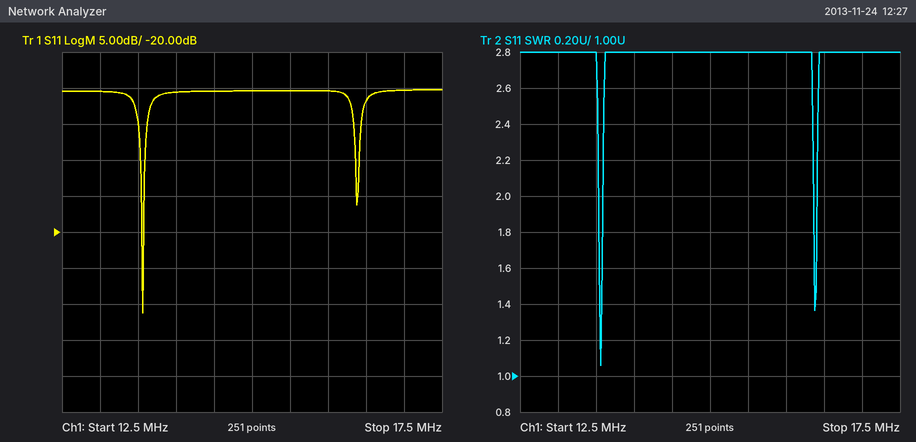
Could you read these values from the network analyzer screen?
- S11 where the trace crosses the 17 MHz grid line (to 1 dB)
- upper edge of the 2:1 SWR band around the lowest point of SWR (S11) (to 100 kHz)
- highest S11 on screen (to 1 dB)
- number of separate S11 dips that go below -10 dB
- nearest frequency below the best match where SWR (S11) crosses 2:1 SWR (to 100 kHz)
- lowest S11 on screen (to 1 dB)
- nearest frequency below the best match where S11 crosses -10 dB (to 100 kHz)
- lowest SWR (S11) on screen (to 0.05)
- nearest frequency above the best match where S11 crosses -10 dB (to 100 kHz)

0 dB
13.6 MHz
0 dB
2
13.5 MHz
-31 dB
13.5 MHz
1.05
13.6 MHz
